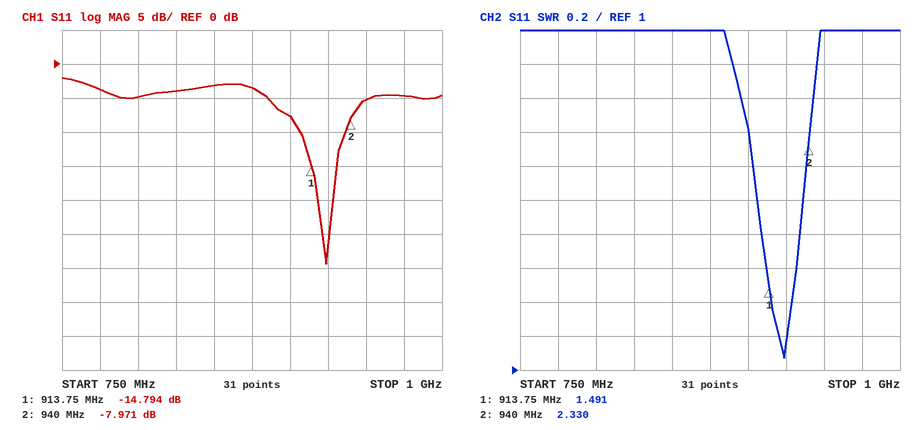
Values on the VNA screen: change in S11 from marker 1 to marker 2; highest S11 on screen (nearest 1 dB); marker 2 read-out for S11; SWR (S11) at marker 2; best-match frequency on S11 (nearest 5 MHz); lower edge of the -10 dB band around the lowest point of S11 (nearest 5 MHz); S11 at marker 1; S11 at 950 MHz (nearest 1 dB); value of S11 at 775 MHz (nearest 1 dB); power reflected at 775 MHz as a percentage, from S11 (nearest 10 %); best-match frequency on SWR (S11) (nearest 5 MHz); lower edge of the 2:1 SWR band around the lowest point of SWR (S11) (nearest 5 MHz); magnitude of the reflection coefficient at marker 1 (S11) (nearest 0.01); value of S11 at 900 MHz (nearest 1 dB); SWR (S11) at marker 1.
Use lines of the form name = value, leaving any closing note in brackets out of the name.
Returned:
change in S11 from marker 1 to marker 2 = 6.823 dB
highest S11 on screen = -2 dB
marker 2 read-out for S11 = -7.971 dB
SWR (S11) at marker 2 = 2.330
best-match frequency on S11 = 925 MHz
lower edge of the -10 dB band around the lowest point of S11 = 905 MHz
S11 at marker 1 = -14.794 dB
S11 at 950 MHz = -5 dB
value of S11 at 775 MHz = -4 dB
power reflected at 775 MHz as a percentage, from S11 = 40 %
best-match frequency on SWR (S11) = 925 MHz
lower edge of the 2:1 SWR band around the lowest point of SWR (S11) = 905 MHz
magnitude of the reflection coefficient at marker 1 (S11) = 0.18
value of S11 at 900 MHz = -8 dB
SWR (S11) at marker 1 = 1.491
